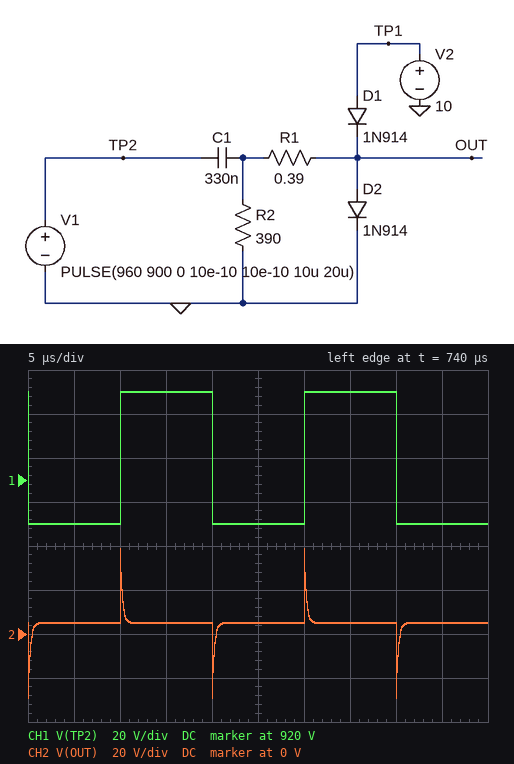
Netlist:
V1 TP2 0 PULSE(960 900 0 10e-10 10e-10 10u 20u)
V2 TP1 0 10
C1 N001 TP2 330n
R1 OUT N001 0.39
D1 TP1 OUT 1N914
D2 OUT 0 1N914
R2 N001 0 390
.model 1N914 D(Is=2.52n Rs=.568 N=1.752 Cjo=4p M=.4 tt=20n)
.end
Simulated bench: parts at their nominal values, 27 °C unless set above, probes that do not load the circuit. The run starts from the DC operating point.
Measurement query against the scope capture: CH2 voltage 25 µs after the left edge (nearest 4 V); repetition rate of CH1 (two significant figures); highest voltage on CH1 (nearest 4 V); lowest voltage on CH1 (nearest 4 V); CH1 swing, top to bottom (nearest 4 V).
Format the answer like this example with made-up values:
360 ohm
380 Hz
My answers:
4 V
50 kHz
960 V
900 V
60 V
